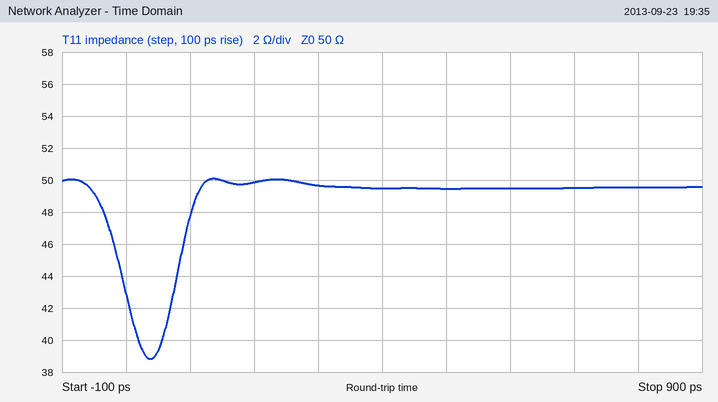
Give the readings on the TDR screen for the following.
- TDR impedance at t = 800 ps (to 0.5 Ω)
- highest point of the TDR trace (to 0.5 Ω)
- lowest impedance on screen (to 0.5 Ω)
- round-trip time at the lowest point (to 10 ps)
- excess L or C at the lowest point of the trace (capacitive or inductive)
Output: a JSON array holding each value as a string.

["49.5 Ω", "50.0 Ω", "39.0 Ω", "40 ps", "capacitive"]
